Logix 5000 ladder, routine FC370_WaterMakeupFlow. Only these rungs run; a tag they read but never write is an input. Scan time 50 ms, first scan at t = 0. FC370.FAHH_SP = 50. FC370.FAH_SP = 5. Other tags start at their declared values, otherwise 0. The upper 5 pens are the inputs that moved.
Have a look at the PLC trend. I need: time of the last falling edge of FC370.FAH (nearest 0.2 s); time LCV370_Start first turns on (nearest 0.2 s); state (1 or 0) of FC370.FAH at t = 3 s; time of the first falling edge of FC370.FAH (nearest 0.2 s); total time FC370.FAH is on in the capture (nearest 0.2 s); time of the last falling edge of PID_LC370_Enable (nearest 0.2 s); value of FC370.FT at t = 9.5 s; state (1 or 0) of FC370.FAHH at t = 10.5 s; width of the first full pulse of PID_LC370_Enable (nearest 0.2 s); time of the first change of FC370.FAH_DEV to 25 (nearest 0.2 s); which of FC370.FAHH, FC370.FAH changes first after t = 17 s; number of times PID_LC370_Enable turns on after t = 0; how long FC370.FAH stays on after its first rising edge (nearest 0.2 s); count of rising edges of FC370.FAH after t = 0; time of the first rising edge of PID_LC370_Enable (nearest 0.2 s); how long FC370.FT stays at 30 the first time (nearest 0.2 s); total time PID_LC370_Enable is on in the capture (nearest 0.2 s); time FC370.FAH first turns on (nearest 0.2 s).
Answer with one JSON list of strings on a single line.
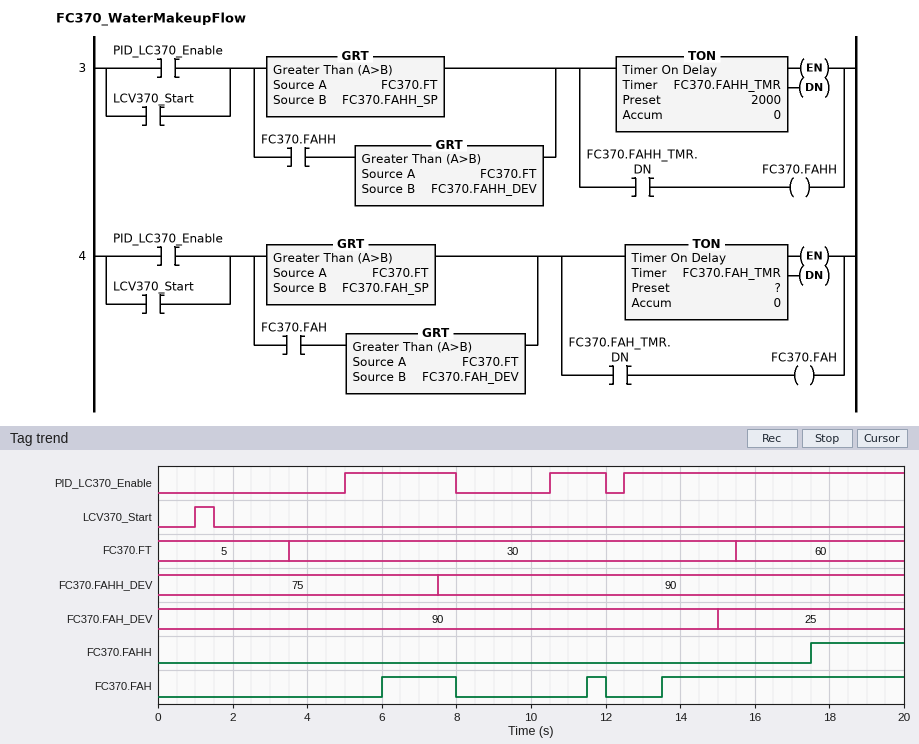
["12.0 s", "1.0 s", "0", "8.0 s", "9.0 s", "12.0 s", "30", "0", "3.0 s", "15.0 s", "FC370.FAHH", "3", "2.0 s", "3", "5.0 s", "12.0 s", "12.0 s", "6.0 s"]
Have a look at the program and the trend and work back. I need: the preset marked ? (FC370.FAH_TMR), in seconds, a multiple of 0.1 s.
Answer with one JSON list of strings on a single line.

["1.0 s"]
